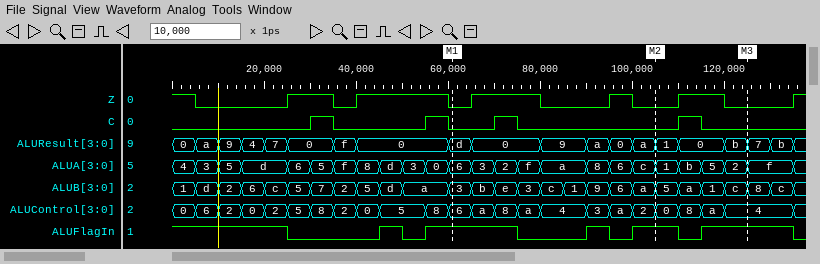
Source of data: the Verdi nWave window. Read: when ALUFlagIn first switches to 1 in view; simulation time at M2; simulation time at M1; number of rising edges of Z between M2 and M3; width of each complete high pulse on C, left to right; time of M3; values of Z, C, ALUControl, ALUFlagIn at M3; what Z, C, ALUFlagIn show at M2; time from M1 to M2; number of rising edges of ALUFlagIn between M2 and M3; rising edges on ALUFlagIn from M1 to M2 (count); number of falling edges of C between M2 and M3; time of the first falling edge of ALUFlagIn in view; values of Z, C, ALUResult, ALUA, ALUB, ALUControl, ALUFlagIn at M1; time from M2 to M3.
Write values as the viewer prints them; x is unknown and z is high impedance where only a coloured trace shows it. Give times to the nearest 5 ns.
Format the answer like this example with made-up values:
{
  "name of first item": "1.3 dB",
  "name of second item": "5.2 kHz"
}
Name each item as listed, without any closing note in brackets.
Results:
{
  "when ALUFlagIn first switches to 1 in view": "45 ns",
  "simulation time at M2": "105 ns",
  "simulation time at M1": "60 ns",
  "number of rising edges of Z between M2 and M3": "1",
  "width of each complete high pulse on C, left to right": "5 ns, 5 ns, 5 ns, 5 ns",
  "time of M3": "125 ns",
  "values of Z, C, ALUControl, ALUFlagIn at M3": "Z=0, C=0, ALUControl=4, ALUFlagIn=1",
  "what Z, C, ALUFlagIn show at M2": "Z=0, C=0, ALUFlagIn=1",
  "time from M1 to M2": "45 ns",
  "number of rising edges of ALUFlagIn between M2 and M3": "1",
  "rising edges on ALUFlagIn from M1 to M2": "2",
  "number of falling edges of C between M2 and M3": "1",
  "time of the first falling edge of ALUFlagIn in view": "25 ns",
  "values of Z, C, ALUResult, ALUA, ALUB, ALUControl, ALUFlagIn at M1": "Z=0, C=0, ALUResult=d, ALUA=6, ALUB=3, ALUControl=6, ALUFlagIn=1",
  "time from M2 to M3": "20 ns"
}
